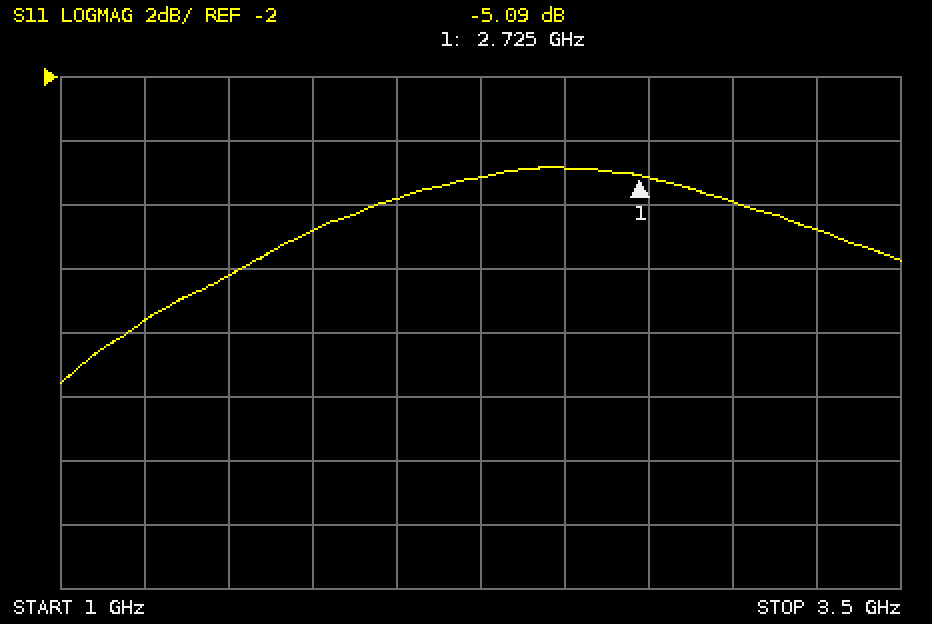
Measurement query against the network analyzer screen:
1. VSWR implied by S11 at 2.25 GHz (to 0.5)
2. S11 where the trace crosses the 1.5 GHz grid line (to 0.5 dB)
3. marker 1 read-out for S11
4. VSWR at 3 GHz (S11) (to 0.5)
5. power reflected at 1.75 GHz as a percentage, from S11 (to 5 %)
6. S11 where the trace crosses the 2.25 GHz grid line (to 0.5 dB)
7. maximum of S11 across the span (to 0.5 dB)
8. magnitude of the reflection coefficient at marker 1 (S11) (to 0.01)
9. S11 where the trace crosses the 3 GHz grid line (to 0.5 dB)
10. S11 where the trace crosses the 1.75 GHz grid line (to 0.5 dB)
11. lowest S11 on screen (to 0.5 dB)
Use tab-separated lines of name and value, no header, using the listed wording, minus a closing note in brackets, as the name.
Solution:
VSWR implied by S11 at 2.25 GHz	3.5
S11 where the trace crosses the 1.5 GHz grid line	-8.0 dB
marker 1 read-out for S11	-5.09 dB
VSWR at 3 GHz (S11)	3.0
power reflected at 1.75 GHz as a percentage, from S11	20 %
S11 where the trace crosses the 2.25 GHz grid line	-5.0 dB
maximum of S11 across the span	-5.0 dB
magnitude of the reflection coefficient at marker 1 (S11)	0.56
S11 where the trace crosses the 3 GHz grid line	-6.0 dB
S11 where the trace crosses the 1.75 GHz grid line	-7.0 dB
lowest S11 on screen	-11.5 dB
